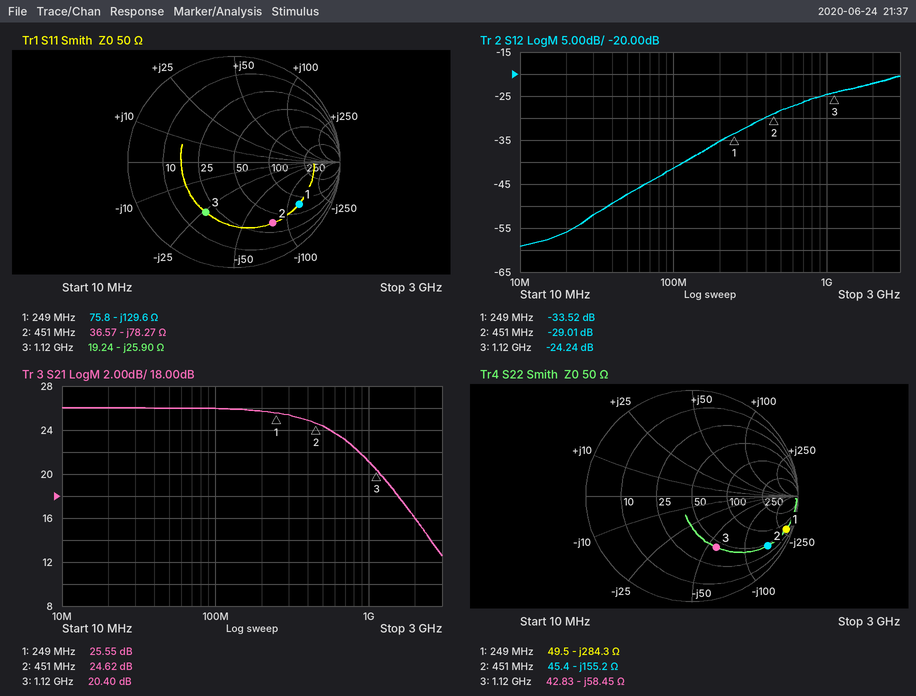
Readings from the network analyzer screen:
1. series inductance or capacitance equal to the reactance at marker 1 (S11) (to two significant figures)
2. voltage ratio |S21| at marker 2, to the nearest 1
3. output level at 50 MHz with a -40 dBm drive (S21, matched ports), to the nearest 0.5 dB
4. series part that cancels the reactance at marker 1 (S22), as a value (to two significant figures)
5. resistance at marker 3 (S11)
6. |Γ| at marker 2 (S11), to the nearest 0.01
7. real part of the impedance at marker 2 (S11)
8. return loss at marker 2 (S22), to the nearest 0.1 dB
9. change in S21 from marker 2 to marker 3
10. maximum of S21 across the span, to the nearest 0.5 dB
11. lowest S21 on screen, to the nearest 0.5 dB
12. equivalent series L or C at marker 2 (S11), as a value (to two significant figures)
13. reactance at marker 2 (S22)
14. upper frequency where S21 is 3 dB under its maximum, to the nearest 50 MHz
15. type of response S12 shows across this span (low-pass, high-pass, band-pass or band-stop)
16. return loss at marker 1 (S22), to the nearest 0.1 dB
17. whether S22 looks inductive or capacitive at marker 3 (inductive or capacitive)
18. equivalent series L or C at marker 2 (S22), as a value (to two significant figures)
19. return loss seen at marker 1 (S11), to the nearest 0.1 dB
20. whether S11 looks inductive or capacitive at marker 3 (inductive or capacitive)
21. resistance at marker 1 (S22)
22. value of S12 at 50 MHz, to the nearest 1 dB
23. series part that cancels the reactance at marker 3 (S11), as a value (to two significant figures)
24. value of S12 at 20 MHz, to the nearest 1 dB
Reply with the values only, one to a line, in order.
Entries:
4.9 pF
17
-14.0 dBm
180 nH
19.24 Ω
0.68
36.57 Ω
1.4 dB
-4.22 dB
26.0 dB
12.5 dB
4.5 pF
-155.2 Ω
700 MHz
high-pass
0.5 dB
capacitive
2.3 pF
2.7 dB
capacitive
49.5 Ω
-47 dB
3.7 nH
-56 dB
